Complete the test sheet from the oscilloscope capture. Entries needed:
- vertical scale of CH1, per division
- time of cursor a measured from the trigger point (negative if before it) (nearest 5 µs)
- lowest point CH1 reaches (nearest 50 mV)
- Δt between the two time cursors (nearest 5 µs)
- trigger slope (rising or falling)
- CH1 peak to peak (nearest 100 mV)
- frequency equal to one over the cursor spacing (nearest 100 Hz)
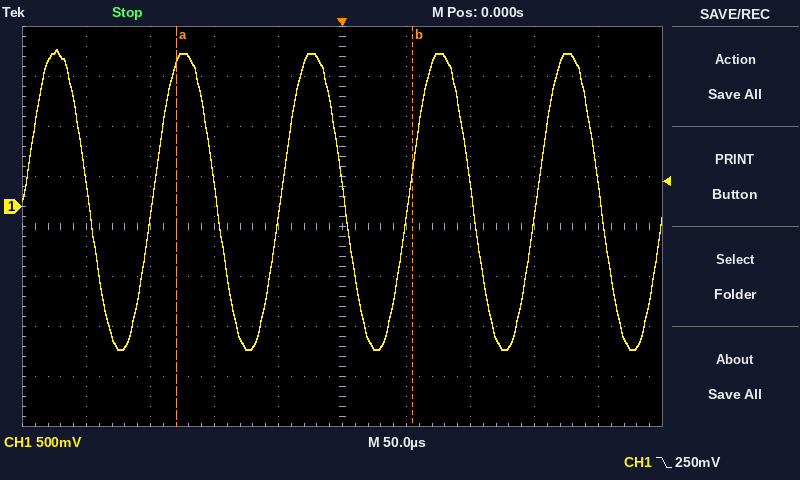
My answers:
500 mV
-130 µs
-1.45 V
185 µs
falling
3.00 V
5.4 kHz
